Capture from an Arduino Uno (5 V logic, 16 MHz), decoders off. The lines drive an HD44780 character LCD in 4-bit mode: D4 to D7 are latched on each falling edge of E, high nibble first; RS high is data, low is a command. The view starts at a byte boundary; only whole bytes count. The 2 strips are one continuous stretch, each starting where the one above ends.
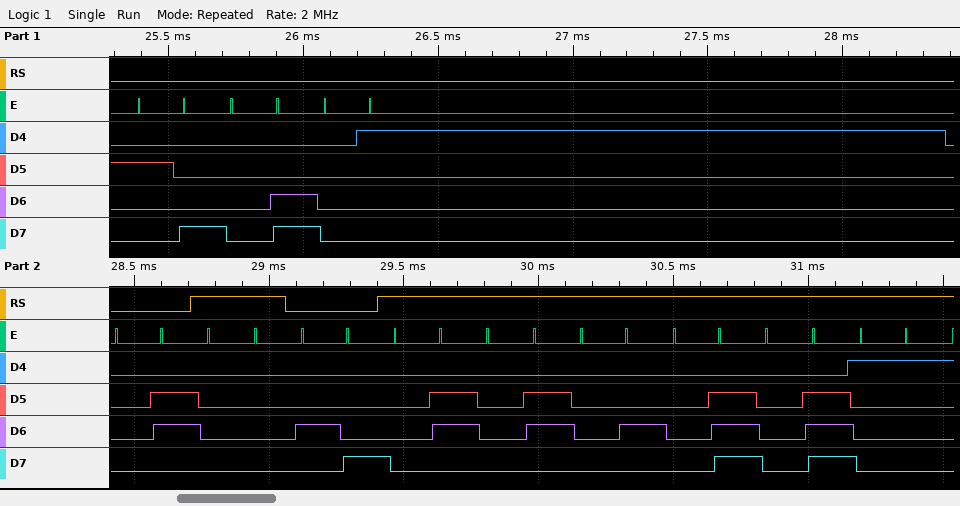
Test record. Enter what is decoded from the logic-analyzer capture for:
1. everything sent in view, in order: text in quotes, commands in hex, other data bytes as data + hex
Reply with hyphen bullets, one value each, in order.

- 0x28 0x0C 0x01 0x06 data 00 0x48 data 06 06 04 0E 0E 11
